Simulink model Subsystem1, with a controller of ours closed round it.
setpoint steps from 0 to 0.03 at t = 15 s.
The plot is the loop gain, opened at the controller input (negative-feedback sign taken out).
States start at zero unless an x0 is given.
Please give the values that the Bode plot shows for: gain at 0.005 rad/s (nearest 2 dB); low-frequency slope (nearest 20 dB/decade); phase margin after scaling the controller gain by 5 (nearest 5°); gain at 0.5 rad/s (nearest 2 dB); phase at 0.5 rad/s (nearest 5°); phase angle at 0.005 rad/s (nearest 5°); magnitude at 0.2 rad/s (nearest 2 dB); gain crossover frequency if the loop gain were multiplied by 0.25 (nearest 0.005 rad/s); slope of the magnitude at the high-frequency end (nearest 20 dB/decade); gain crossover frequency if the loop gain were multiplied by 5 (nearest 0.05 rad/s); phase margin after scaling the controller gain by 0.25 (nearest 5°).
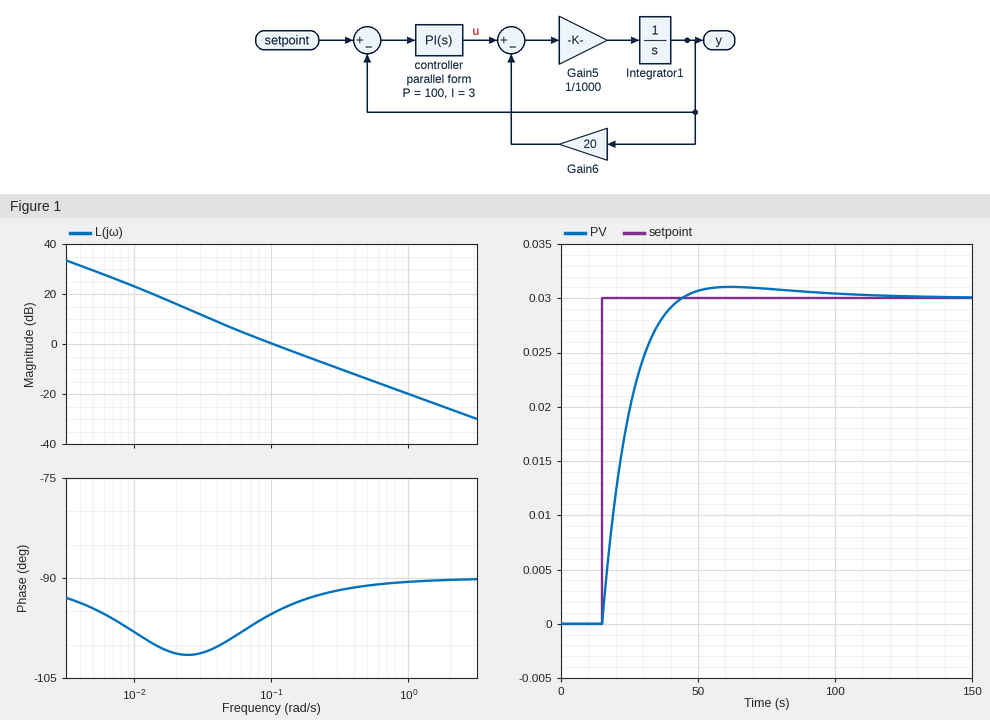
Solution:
30 dB
-20 dB/decade
90°
-14 dB
-90°
-95°
-6 dB
0.030 rad/s
-20 dB/decade
0.50 rad/s
80°
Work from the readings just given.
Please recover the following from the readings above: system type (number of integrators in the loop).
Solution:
1
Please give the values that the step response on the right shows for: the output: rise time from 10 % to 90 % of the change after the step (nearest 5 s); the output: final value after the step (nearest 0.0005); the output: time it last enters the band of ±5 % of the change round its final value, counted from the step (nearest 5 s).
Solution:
20 s
0.0300
25 s
